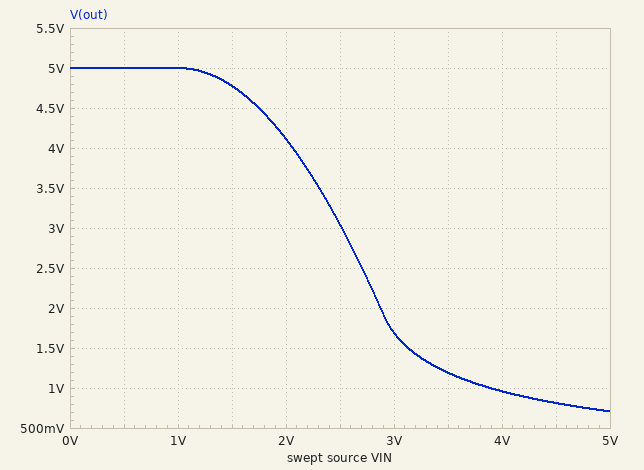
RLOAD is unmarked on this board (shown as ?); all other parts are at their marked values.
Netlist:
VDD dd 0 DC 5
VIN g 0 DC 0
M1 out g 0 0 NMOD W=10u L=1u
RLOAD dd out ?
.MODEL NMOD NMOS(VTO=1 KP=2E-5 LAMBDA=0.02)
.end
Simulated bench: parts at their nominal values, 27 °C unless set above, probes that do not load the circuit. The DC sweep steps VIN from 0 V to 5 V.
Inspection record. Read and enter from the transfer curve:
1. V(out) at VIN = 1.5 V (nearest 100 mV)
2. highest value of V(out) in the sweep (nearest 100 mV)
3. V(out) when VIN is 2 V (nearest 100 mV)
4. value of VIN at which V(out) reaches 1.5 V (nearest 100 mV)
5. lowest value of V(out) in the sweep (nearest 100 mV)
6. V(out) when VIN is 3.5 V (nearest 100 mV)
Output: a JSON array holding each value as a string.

["4.8 V", "5.0 V", "4.1 V", "3.1 V", "700 mV", "1.2 V"]
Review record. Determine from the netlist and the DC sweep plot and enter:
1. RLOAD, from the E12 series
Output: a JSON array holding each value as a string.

["8.2 kΩ"]
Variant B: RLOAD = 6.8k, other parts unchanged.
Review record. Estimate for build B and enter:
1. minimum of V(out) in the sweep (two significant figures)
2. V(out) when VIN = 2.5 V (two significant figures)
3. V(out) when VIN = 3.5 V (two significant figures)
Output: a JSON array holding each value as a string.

["840 mV", "3.4 V", "1.4 V"]
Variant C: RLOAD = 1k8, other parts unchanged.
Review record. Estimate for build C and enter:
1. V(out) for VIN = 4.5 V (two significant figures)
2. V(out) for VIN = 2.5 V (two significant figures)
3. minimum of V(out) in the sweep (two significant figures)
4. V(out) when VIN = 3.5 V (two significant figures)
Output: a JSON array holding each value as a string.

["2.8 V", "4.6 V", "2.4 V", "3.8 V"]
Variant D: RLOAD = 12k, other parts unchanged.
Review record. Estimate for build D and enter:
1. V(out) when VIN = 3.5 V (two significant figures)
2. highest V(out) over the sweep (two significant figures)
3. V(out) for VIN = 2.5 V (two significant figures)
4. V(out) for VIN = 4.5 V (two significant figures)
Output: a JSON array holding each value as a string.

["820 mV", "5.0 V", "2.2 V", "570 mV"]
